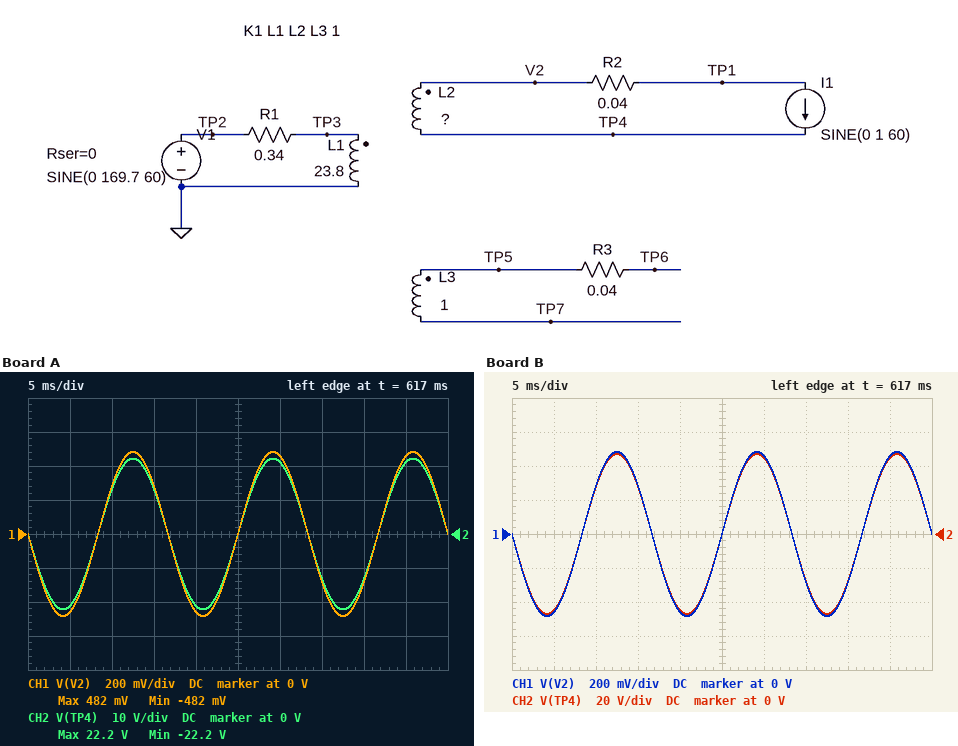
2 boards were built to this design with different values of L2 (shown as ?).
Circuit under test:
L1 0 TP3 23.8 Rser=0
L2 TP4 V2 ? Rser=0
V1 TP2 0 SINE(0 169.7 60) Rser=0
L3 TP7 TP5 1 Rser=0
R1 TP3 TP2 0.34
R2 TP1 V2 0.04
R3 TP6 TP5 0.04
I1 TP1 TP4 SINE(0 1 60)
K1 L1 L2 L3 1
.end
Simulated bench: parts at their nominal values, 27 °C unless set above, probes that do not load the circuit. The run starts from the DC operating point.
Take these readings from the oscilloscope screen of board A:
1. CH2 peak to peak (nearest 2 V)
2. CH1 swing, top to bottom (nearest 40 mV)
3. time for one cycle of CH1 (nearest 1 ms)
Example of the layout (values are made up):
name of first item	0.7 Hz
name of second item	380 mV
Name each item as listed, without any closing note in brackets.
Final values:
CH2 peak to peak	44 V
CH1 swing, top to bottom	960 mV
time for one cycle of CH1	17 ms
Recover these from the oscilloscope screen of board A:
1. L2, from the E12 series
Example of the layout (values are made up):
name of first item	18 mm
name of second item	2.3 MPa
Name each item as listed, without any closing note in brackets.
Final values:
L2, from the E12 series	390 mH
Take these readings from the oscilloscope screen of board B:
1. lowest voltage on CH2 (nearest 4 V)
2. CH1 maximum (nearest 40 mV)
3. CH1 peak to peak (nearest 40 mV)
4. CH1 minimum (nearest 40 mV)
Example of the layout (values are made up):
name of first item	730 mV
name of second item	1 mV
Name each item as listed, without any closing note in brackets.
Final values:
lowest voltage on CH2	-48 V
CH1 maximum	480 mV
CH1 peak to peak	960 mV
CH1 minimum	-480 mV
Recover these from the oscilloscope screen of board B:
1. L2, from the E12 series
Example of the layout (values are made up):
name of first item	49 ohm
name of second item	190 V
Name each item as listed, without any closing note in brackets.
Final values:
L2, from the E12 series	1.8 H
